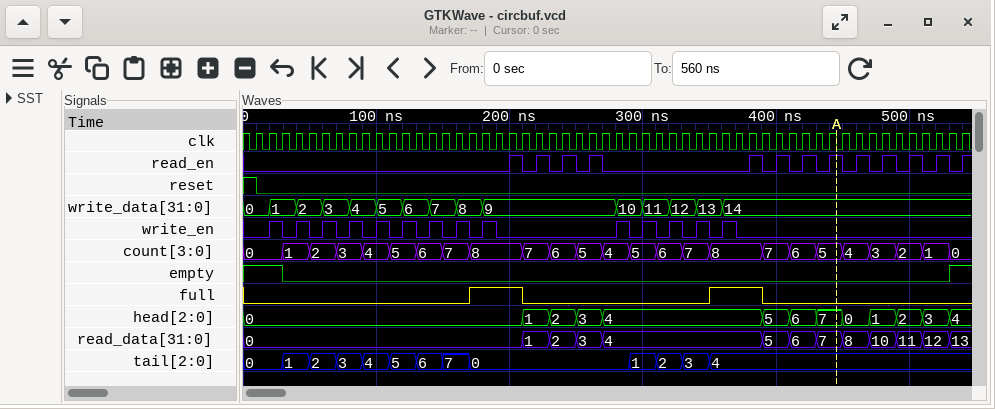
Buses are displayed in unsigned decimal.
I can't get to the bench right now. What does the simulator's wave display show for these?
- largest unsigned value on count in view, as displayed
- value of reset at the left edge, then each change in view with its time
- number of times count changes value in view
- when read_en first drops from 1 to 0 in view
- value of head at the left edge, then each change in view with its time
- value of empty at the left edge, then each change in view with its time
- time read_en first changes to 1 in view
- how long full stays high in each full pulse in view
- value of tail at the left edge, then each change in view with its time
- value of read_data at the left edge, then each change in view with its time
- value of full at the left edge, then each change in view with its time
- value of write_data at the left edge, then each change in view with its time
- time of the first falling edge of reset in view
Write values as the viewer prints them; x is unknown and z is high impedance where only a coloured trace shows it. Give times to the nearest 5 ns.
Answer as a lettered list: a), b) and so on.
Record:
a) 8
b) 1, 0 at 10 ns
c) 24
d) 210 ns
e) 0, 1 at 210 ns, 2 at 230 ns, 3 at 250 ns, 4 at 270 ns, 5 at 390 ns, 6 at 410 ns, 7 at 430 ns, 0 at 450 ns, 1 at 470 ns, 2 at 490 ns, 3 at 510 ns, 4 at 530 ns
f) 1, 0 at 30 ns, 1 at 530 ns
g) 200 ns
h) 40 ns, 40 ns
i) 0, 1 at 30 ns, 2 at 50 ns, 3 at 70 ns, 4 at 90 ns, 5 at 110 ns, 6 at 130 ns, 7 at 150 ns, 0 at 170 ns, 1 at 290 ns, 2 at 310 ns, 3 at 330 ns, 4 at 350 ns
j) 0, 1 at 210 ns, 2 at 230 ns, 3 at 250 ns, 4 at 270 ns, 5 at 390 ns, 6 at 410 ns, 7 at 430 ns, 8 at 450 ns, 10 at 470 ns, 11 at 490 ns, 12 at 510 ns, 13 at 530 ns
k) 0, 1 at 170 ns, 0 at 210 ns, 1 at 350 ns, 0 at 390 ns
l) 0, 1 at 20 ns, 2 at 40 ns, 3 at 60 ns, 4 at 80 ns, 5 at 100 ns, 6 at 120 ns, 7 at 140 ns, 8 at 160 ns, 9 at 180 ns, 10 at 280 ns, 11 at 300 ns, 12 at 320 ns, 13 at 340 ns, 14 at 360 ns
m) 10 ns
